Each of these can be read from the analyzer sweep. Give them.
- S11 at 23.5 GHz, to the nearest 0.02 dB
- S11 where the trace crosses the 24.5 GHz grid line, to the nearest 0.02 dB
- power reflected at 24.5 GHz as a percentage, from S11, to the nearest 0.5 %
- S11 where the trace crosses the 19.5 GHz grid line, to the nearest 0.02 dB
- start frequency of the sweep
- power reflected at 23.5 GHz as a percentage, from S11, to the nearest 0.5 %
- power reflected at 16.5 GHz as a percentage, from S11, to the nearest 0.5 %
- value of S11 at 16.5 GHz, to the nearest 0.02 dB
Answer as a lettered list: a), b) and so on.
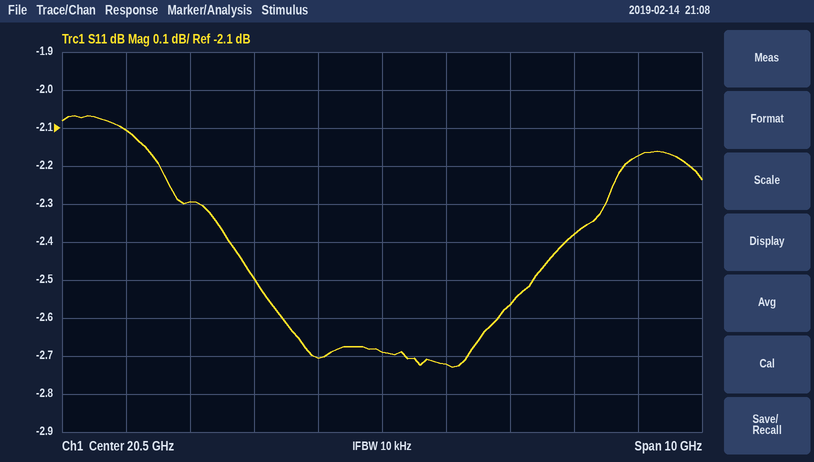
a) -2.38 dB
b) -2.18 dB
c) 60.5 %
d) -2.70 dB
e) 15.5 GHz
f) 58.0 %
g) 61.5 %
h) -2.10 dB
